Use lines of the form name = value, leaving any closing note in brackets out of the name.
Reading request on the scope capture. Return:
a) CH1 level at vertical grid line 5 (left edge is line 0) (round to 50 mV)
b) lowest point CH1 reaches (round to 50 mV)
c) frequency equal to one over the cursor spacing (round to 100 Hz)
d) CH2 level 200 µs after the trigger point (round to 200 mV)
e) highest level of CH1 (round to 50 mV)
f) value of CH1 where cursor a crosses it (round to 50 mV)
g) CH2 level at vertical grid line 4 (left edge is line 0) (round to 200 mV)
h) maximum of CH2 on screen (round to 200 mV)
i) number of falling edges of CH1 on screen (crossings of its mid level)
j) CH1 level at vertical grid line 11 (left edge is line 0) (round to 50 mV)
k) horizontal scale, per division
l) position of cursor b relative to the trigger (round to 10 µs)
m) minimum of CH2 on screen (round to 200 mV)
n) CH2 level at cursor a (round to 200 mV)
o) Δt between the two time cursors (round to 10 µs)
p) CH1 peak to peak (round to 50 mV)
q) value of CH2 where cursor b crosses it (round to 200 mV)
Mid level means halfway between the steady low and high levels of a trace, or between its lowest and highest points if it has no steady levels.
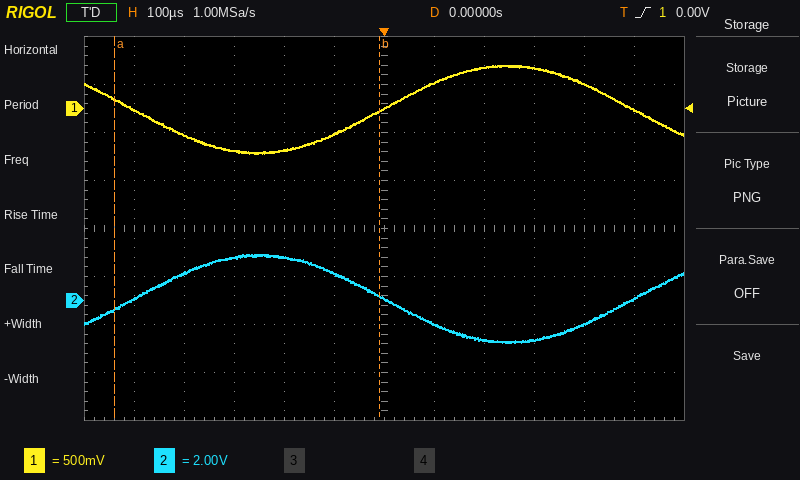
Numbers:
CH1 level at vertical grid line 5 (left edge is line 0) = -250 mV
lowest point CH1 reaches = -450 mV
frequency equal to one over the cursor spacing = 1.9 kHz
CH2 level 200 µs after the trigger point = -1.6 V
highest level of CH1 = 450 mV
value of CH1 where cursor a crosses it = 100 mV
CH2 level at vertical grid line 4 (left edge is line 0) = 1.8 V
maximum of CH2 on screen = 2.0 V
number of falling edges of CH1 on screen = 2
CH1 level at vertical grid line 11 (left edge is line 0) = 0 mV
horizontal scale, per division = 100 µs
position of cursor b relative to the trigger = -10 µs
minimum of CH2 on screen = -1.8 V
CH2 level at cursor a = -400 mV
Δt between the two time cursors = 530 µs
CH1 peak to peak = 900 mV
value of CH2 where cursor b crosses it = 200 mV
